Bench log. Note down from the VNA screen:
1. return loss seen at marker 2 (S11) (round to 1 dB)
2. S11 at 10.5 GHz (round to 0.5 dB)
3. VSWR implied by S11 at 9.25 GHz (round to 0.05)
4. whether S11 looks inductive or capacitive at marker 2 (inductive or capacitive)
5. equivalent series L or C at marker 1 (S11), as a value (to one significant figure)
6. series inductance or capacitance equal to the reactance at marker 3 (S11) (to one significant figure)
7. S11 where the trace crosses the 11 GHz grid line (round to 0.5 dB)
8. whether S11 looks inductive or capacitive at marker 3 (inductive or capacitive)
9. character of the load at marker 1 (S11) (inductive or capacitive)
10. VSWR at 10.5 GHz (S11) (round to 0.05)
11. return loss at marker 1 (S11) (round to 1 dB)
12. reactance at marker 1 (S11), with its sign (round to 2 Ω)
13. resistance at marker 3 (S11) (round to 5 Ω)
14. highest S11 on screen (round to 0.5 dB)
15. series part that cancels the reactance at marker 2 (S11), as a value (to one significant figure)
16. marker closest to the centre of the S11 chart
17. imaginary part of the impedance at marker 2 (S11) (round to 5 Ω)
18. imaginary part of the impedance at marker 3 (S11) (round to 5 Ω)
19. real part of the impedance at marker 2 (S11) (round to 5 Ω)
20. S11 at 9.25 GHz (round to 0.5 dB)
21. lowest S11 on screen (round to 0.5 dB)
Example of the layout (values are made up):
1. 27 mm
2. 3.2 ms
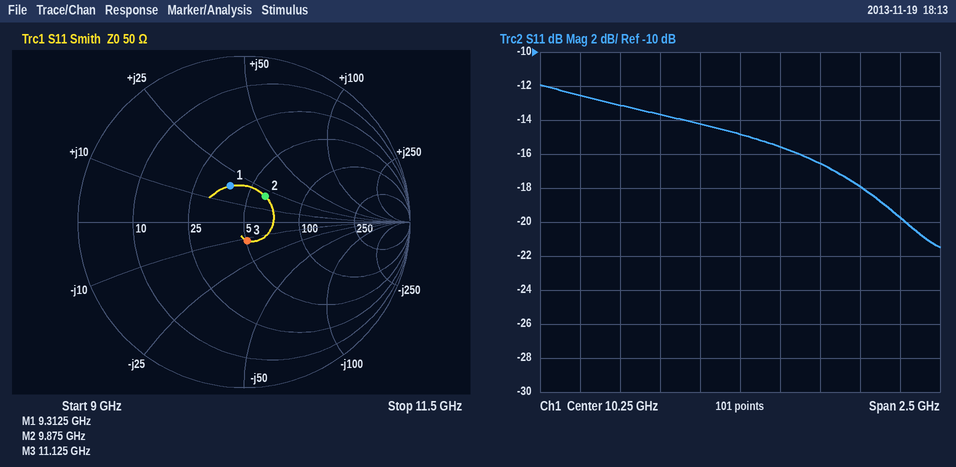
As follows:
1. 14 dB
2. -15.5 dB
3. 1.60
4. inductive
5. 300 pH
6. 1 pF
7. -18.0 dB
8. capacitive
9. inductive
10. 1.40
11. 13 dB
12. +18 Ω
13. 50 Ω
14. -12.0 dB
15. 800 fF
16. marker 3
17. +20 Ω
18. -10 Ω
19. 60 Ω
20. -12.5 dB
21. -21.5 dB
